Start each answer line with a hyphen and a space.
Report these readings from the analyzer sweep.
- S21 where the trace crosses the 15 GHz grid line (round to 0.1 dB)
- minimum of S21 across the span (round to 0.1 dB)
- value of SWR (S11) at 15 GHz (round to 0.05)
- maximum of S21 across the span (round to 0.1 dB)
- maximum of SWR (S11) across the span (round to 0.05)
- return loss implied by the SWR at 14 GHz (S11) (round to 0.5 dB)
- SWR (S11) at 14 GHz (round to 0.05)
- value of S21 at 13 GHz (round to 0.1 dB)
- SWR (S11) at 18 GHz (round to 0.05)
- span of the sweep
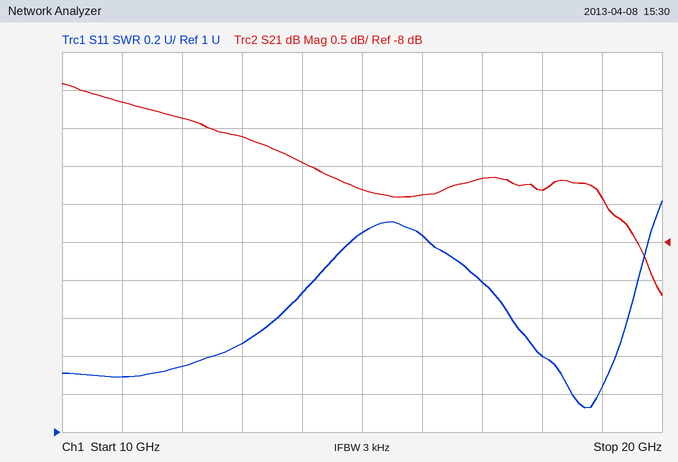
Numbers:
- -7.3 dB
- -8.7 dB
- 2.05
- -5.9 dB
- 2.20
- 11.5 dB
- 1.75
- -6.6 dB
- 1.40
- 10 GHz
